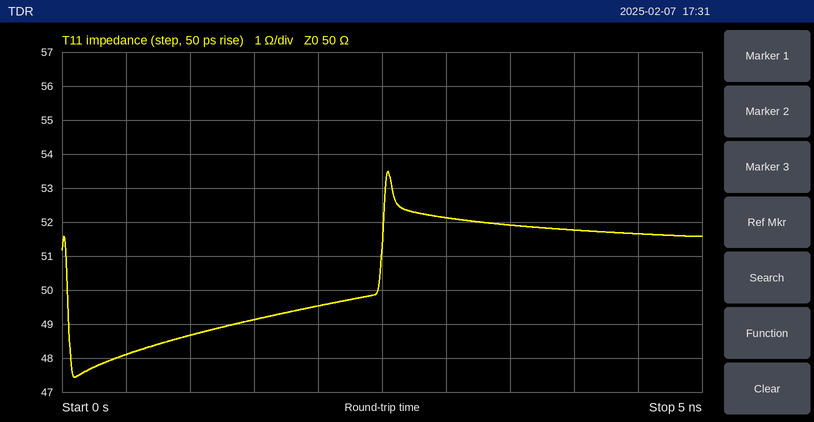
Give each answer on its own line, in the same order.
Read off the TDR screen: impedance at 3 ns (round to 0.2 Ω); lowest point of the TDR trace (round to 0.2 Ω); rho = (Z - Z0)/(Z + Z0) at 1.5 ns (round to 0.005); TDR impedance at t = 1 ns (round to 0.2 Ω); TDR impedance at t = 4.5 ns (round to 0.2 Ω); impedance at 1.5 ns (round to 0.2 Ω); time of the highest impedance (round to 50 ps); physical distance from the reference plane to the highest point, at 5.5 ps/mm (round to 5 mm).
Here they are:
52.2 Ω
47.4 Ω
-0.010
48.6 Ω
51.6 Ω
49.2 Ω
2.55 ns
230 mm
